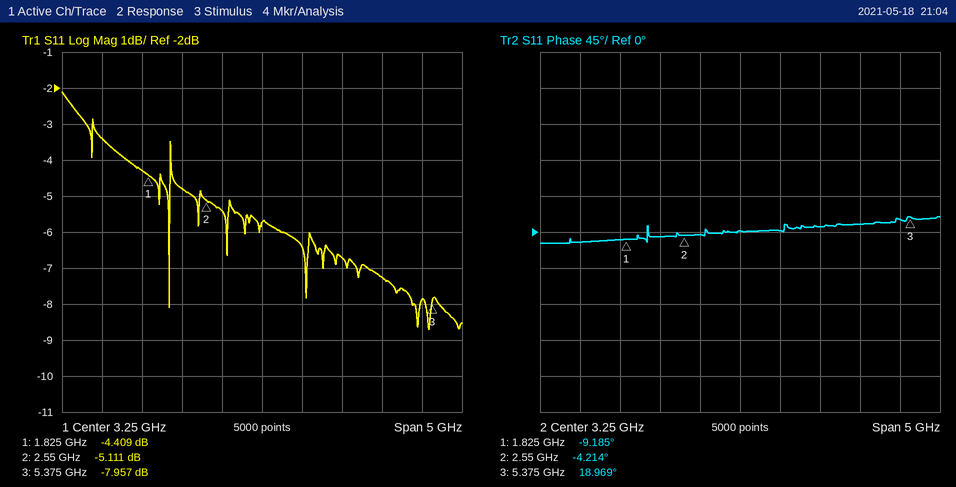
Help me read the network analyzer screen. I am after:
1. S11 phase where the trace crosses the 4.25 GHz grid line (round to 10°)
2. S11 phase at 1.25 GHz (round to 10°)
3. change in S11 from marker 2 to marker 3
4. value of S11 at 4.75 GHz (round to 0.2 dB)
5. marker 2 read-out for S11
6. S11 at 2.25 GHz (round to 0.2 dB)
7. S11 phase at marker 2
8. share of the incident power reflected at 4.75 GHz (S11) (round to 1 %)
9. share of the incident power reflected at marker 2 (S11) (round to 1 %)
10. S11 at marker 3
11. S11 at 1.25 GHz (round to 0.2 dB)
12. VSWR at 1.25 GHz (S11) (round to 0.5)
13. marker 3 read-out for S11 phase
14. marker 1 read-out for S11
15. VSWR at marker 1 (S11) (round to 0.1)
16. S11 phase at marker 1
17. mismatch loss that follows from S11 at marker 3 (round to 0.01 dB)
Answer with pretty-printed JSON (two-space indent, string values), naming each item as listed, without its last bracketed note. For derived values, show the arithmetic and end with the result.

{
  "S11 phase where the trace crosses the 4.25 GHz grid line": "10°",
  "S11 phase at 1.25 GHz": "-10°",
  "change in S11 from marker 2 to marker 3": "-7.957 − (-5.111) = -2.846 dB",
  "value of S11 at 4.75 GHz": "-7.2 dB",
  "marker 2 read-out for S11": "-5.111 dB",
  "S11 at 2.25 GHz": "-4.8 dB",
  "S11 phase at marker 2": "-4.214°",
  "share of the incident power reflected at 4.75 GHz (S11)": "10^(-7.2/10) ≈ 19 %",
  "share of the incident power reflected at marker 2 (S11)": "10^(-5.111/10) ≈ 31 %",
  "S11 at marker 3": "-7.957 dB",
  "S11 at 1.25 GHz": "-3.4 dB",
  "VSWR at 1.25 GHz (S11)": "|Γ| = 10^(-3.4/20) = 0.6761; VSWR = (1 + 0.6761)/(1 − 0.6761) ≈ 5.17, so 5.0 to the nearest 0.5",
  "marker 3 read-out for S11 phase": "18.969°",
  "marker 1 read-out for S11": "-4.409 dB",
  "VSWR at marker 1 (S11)": "(1 + 0.6019)/(1 − 0.6019) ≈ 4.0",
  "S11 phase at marker 1": "-9.185°",
  "mismatch loss that follows from S11 at marker 3": "−10 log10(1 − 10^(-7.957/10)) ≈ 0.76 dB"
}
